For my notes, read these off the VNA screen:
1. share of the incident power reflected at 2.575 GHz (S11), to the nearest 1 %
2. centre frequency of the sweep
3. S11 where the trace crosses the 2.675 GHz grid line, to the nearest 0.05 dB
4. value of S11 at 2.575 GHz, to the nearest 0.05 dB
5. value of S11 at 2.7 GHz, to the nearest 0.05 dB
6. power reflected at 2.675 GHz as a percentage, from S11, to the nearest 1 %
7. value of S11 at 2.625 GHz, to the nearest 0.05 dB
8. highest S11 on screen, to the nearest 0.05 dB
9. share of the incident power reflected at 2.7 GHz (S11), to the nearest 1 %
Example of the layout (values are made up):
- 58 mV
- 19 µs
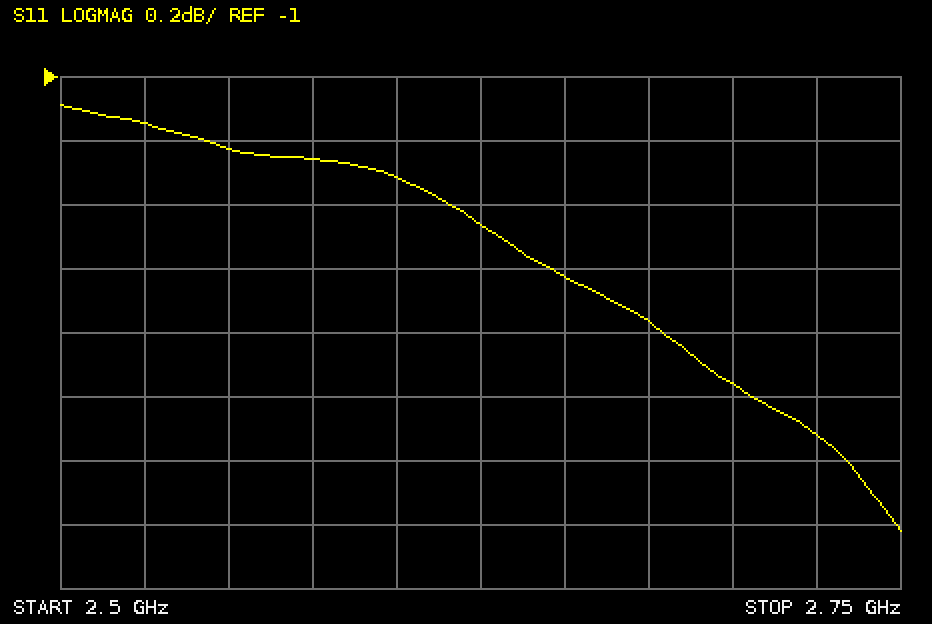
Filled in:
- 75 %
- 2.625 GHz
- -1.75 dB
- -1.25 dB
- -1.95 dB
- 67 %
- -1.45 dB
- -1.10 dB
- 64 %
